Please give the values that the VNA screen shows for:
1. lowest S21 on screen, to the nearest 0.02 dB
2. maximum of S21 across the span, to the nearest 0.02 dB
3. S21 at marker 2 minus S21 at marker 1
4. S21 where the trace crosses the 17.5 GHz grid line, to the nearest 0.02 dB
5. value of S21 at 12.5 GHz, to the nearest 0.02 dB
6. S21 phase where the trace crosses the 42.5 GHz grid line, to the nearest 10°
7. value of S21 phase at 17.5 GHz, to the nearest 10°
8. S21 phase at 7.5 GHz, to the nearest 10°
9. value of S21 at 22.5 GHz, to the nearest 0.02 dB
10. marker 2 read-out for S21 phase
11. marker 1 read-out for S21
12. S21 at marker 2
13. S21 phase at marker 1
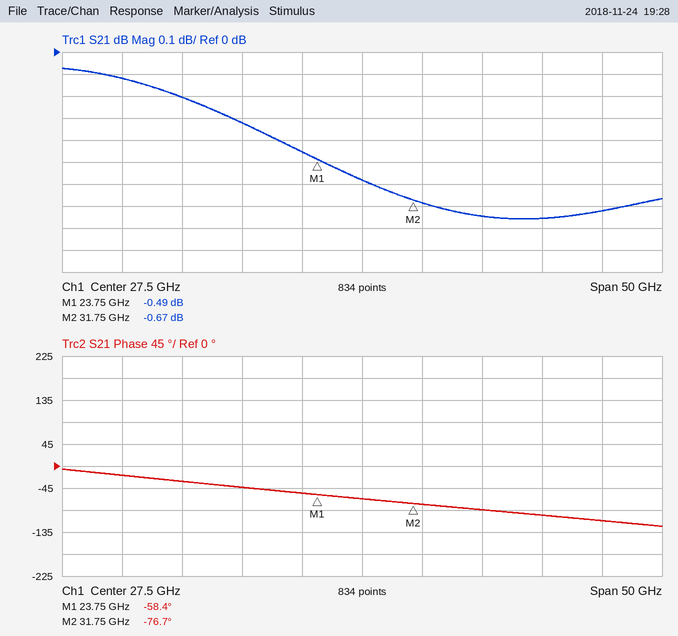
-0.76 dB
-0.08 dB
-0.18 dB
-0.32 dB
-0.20 dB
-100°
-40°
-20°
-0.46 dB
-76.7°
-0.49 dB
-0.67 dB
-58.4°
